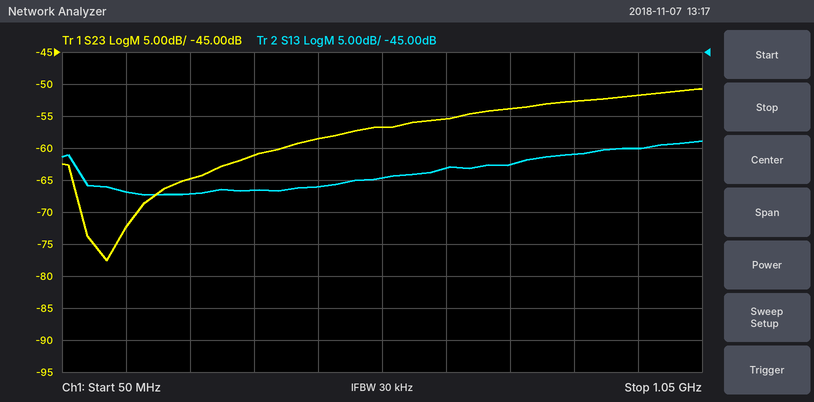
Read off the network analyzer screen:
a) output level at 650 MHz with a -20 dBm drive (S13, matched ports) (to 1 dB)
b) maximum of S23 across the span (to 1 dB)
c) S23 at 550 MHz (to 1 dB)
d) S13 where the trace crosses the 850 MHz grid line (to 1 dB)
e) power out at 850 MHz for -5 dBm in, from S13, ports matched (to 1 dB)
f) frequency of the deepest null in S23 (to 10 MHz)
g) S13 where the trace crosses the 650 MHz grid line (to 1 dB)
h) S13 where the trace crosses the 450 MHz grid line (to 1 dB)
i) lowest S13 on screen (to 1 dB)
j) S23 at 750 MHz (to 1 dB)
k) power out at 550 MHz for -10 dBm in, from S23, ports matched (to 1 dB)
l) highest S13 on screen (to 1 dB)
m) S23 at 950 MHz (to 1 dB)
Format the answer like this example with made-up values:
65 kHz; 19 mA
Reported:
-83 dBm; -51 dB; -57 dB; -61 dB; -66 dBm; 120 MHz; -63 dB; -66 dB; -67 dB; -54 dB; -67 dBm; -59 dB; -52 dB
